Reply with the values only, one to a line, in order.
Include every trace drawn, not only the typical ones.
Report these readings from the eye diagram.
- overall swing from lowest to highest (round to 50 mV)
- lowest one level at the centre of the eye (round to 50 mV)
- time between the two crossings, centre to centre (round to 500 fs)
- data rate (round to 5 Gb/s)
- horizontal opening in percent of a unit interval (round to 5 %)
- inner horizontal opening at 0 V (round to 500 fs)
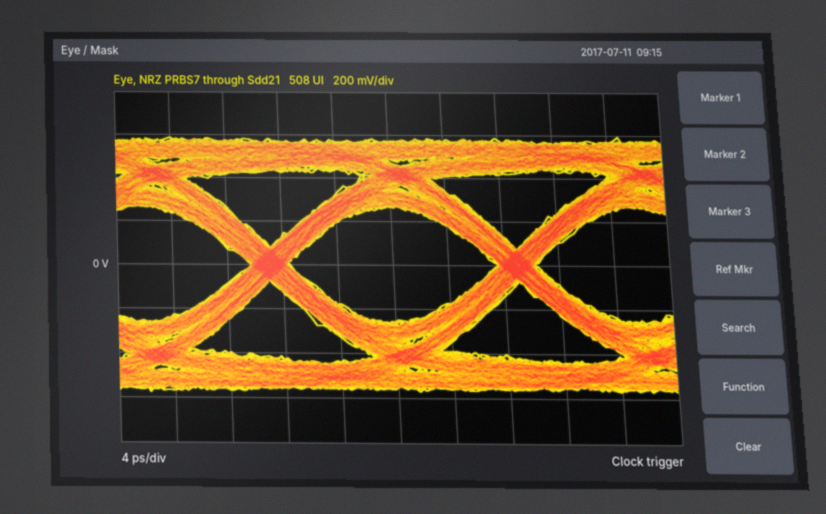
1.15 V
250 mV
18.0 ps
55 Gb/s
85 %
15.0 ps
